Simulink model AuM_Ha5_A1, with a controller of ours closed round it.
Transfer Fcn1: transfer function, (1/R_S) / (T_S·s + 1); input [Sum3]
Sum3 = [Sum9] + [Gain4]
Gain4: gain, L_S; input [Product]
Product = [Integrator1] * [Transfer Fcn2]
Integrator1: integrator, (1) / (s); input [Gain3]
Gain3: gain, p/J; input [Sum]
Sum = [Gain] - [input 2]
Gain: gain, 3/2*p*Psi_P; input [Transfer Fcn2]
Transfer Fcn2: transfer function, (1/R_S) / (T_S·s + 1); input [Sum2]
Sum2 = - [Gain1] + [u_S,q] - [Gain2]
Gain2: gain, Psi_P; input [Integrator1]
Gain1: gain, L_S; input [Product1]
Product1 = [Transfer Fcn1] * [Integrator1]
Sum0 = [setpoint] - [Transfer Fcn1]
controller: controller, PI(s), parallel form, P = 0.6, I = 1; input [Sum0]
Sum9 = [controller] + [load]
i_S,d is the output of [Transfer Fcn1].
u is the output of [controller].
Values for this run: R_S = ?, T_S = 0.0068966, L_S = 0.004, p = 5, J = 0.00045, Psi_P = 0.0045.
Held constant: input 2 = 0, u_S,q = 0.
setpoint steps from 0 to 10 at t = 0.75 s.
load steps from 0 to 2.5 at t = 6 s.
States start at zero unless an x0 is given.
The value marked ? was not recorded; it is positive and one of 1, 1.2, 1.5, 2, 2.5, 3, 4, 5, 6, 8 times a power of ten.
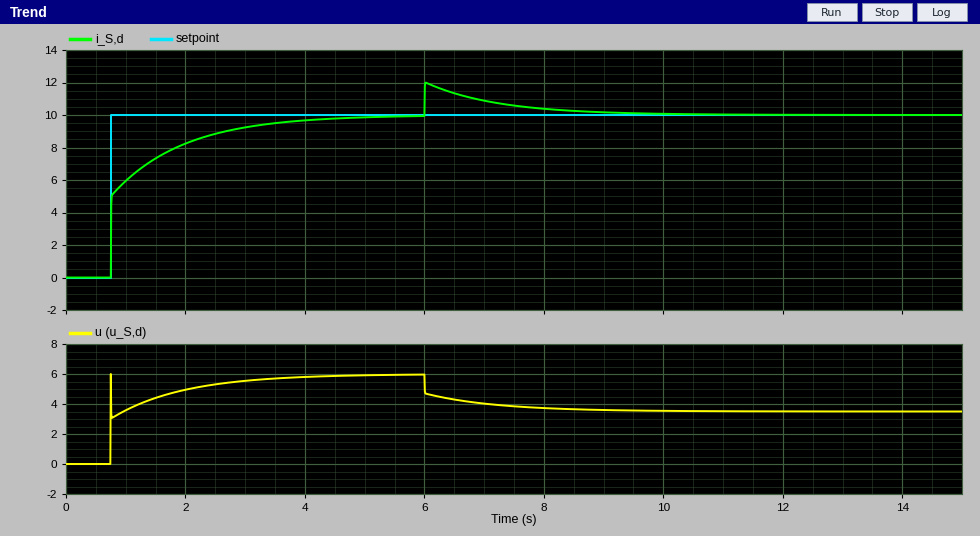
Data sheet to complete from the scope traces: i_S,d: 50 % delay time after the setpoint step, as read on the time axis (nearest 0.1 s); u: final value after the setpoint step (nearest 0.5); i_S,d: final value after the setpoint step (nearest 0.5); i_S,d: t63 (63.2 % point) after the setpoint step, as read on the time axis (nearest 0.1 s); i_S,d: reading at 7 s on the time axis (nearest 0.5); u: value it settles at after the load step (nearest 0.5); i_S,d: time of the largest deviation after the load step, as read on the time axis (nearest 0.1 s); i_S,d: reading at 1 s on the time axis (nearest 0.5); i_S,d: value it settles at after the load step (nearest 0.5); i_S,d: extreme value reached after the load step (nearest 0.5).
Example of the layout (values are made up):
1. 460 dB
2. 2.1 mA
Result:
1. 0.8 s
2. 6.0
3. 10.0
4. 1.1 s
5. 11.0
6. 3.5
7. 6.0 s
8. 6.0
9. 10.0
10. 12.0
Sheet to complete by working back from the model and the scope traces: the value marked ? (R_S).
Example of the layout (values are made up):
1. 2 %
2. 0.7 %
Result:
1. 0.6
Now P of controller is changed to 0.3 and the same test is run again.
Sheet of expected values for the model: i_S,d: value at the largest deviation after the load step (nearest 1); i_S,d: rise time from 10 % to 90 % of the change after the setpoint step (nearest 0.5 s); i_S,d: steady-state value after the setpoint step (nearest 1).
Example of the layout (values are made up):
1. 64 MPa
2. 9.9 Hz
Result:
1. 13
2. 1.5 s
3. 10
